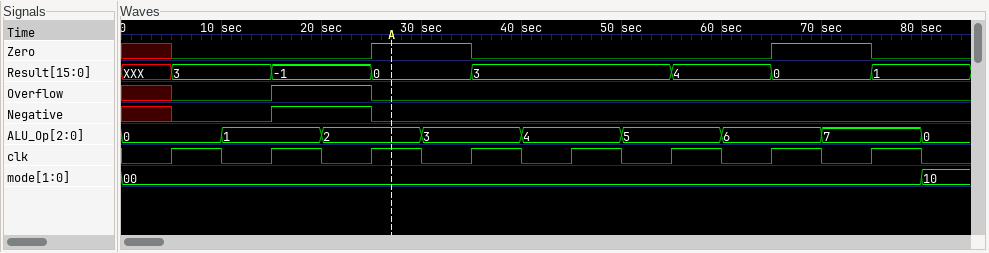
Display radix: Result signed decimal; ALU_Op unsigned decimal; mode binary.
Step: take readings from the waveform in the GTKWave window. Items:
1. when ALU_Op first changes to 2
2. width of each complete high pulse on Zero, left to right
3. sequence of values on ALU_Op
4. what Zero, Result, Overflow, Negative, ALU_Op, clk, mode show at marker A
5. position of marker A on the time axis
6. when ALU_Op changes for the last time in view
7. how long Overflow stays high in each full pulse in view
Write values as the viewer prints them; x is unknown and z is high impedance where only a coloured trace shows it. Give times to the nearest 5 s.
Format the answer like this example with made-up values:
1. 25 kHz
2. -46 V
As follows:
1. 20 s
2. 10 s, 10 s
3. 0, 1, 2, 3, 4, 5, 6, 7, 0
4. Zero=1, Result=0, Overflow=0, Negative=0, ALU_Op=2, clk=1, mode=00
5. 25 s
6. 80 s
7. 10 s
